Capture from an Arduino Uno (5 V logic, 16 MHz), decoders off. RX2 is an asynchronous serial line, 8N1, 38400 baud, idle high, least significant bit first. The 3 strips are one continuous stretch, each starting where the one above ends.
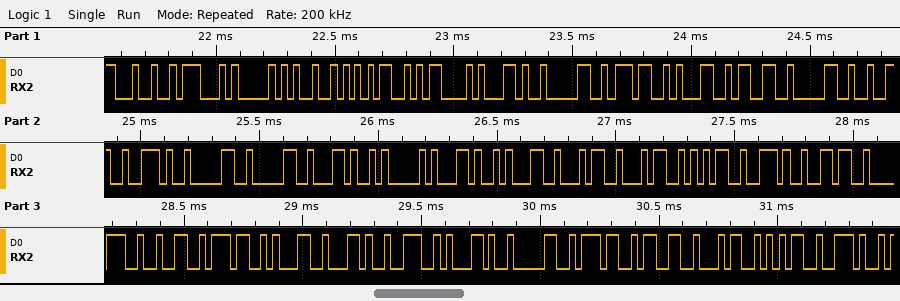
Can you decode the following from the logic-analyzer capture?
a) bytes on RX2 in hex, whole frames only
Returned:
24 47 50 52 4D 43 2C 30 37 31 33 30 32 2E 30 30 2C 41 2C 31 34 34 35 2E 36 38 32 37 31 2C 4E 2C 30 37 33 34 35 2E
